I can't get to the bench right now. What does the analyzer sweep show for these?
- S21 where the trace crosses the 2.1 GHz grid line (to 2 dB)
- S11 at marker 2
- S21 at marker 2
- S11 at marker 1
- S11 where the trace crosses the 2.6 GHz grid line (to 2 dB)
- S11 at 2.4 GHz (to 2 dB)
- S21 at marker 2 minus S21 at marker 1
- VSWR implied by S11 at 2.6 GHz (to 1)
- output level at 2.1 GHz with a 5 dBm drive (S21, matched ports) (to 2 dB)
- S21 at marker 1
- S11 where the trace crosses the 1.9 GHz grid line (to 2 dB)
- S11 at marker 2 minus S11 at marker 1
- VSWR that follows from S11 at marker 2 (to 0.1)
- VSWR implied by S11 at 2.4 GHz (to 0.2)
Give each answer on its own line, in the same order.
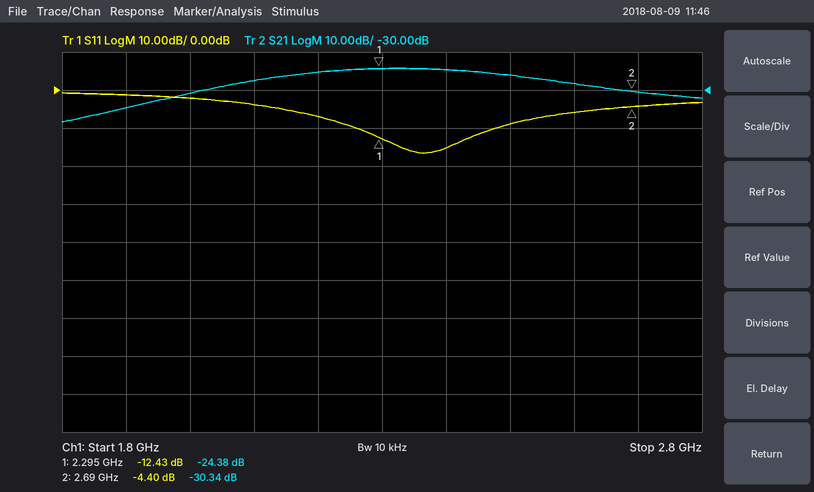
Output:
-28 dB
-4.40 dB
-30.34 dB
-12.43 dB
-6 dB
-16 dB
-5.96 dB
3
-22 dBm
-24.38 dB
-2 dB
8.03 dB
4.0
1.4
